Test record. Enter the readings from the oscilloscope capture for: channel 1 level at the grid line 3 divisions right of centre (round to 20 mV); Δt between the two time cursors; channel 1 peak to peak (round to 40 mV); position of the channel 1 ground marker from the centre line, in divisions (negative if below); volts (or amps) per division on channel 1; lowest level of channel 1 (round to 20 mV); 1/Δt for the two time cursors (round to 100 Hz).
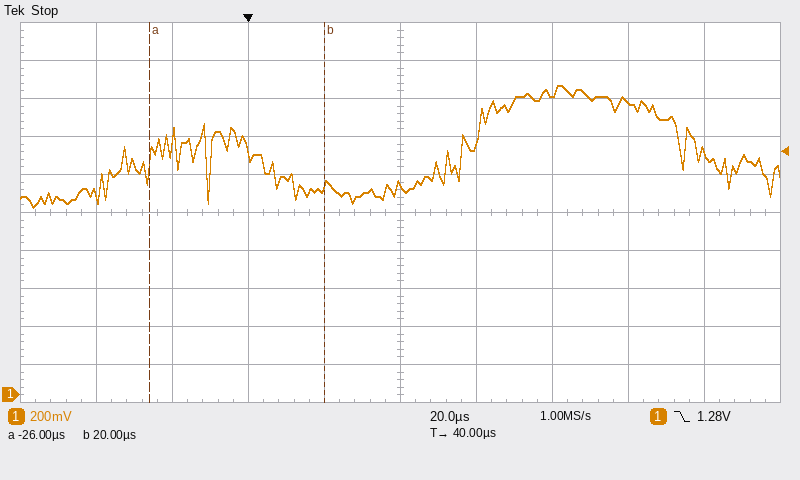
1.54 V
46 µs
640 mV
-4.8 div
200 mV
980 mV
21.7 kHz
